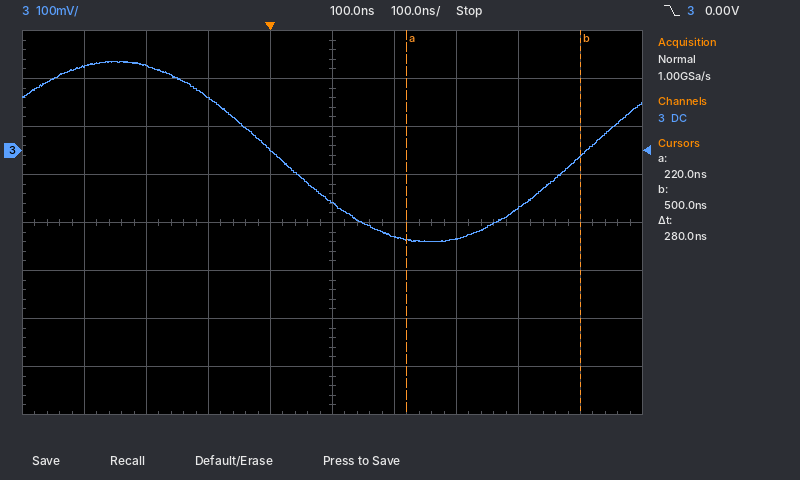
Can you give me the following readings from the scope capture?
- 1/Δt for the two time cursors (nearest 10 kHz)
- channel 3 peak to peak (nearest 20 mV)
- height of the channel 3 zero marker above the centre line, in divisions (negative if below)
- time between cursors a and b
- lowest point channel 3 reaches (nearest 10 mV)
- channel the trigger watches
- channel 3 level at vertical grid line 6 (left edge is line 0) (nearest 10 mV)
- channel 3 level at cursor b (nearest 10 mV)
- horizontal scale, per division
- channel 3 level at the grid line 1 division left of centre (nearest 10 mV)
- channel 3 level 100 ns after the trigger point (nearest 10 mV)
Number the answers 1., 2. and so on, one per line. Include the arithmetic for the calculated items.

1. 1 / 280 ns ≈ 3.57 MHz
2. 380 mV
3. +1.5 div
4. 280 ns
5. -190 mV
6. channel 3
7. -180 mV
8. -10 mV
9. 100 ns
10. 0 mV
11. -110 mV
